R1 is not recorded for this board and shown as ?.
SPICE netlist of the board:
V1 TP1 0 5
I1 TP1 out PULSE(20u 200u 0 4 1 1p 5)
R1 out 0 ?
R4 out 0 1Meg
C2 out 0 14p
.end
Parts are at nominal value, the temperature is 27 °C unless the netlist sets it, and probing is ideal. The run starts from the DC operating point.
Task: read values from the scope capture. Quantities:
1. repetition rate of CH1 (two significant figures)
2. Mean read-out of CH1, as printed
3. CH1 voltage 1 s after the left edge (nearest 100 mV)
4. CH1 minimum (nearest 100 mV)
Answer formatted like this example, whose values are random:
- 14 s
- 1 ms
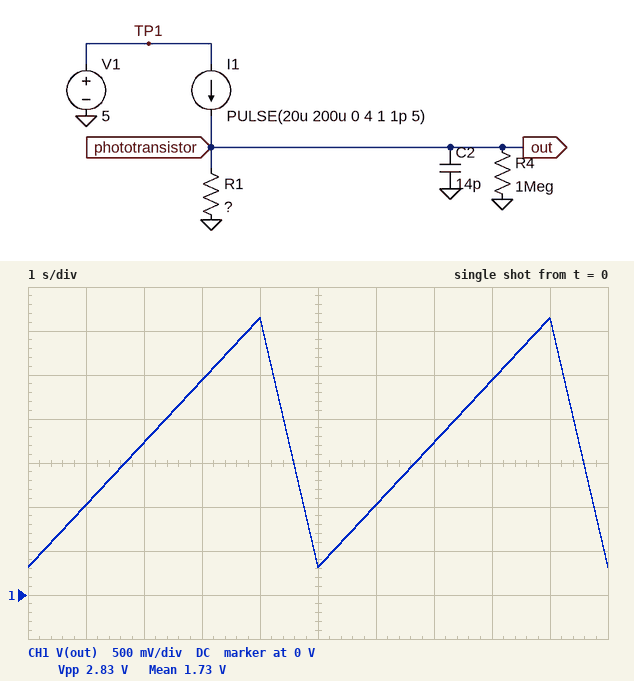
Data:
- 200 mHz
- 1.73 V
- 1.0 V
- 300 mV
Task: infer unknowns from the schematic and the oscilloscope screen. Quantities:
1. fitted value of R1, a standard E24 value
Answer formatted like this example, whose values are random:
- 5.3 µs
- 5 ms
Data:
- 16 kΩ
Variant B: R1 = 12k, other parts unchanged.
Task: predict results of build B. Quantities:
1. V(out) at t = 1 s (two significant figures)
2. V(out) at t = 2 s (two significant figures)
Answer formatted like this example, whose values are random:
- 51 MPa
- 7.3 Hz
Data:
- 770 mV
- 1.3 V
